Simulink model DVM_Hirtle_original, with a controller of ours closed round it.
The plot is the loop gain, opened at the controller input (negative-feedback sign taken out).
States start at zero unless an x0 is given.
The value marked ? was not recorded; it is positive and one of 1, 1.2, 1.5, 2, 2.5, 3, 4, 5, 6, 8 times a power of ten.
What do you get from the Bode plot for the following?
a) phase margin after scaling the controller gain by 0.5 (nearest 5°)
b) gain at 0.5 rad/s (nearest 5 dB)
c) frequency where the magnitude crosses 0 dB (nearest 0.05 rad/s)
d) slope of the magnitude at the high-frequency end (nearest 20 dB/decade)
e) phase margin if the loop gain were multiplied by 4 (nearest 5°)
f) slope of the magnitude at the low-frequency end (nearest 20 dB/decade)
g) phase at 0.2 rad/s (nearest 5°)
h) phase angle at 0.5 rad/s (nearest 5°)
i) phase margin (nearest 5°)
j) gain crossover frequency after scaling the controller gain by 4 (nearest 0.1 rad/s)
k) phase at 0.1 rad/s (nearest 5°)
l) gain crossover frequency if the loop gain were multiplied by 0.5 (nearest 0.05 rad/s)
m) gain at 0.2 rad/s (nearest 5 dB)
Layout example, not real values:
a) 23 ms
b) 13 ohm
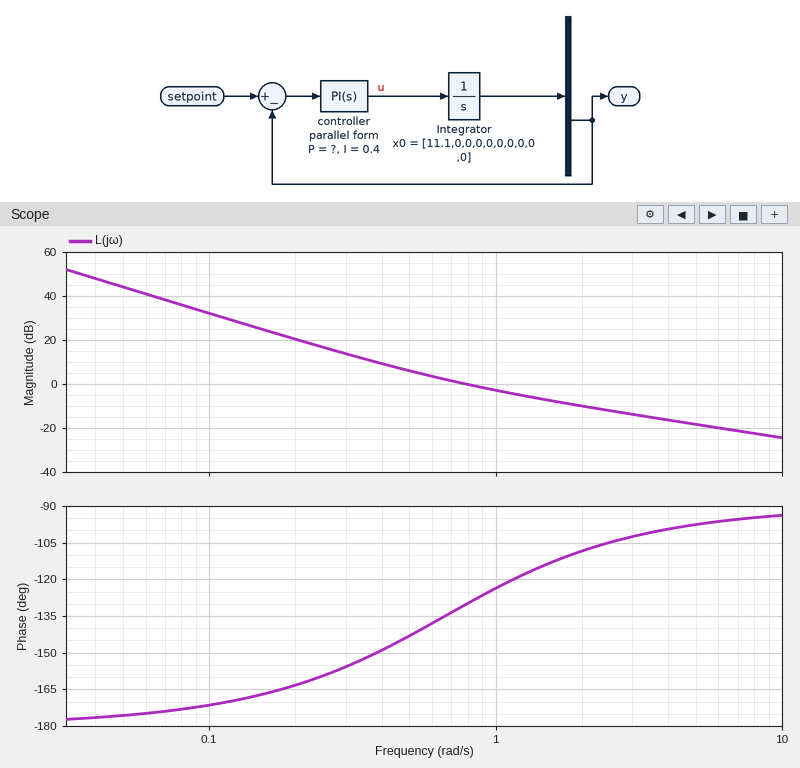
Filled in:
a) 35°
b) 5 dB
c) 0.80 rad/s
d) -20 dB/decade
e) 75°
f) -40 dB/decade
g) -165°
h) -145°
i) 50°
j) 2.5 rad/s
k) -170°
l) 0.50 rad/s
m) 20 dB
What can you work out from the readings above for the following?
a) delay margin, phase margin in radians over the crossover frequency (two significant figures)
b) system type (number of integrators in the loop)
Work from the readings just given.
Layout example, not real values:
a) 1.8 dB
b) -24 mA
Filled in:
a) 1.1 s
b) 2
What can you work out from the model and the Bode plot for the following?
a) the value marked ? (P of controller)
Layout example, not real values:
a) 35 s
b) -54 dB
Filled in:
a) 0.6
